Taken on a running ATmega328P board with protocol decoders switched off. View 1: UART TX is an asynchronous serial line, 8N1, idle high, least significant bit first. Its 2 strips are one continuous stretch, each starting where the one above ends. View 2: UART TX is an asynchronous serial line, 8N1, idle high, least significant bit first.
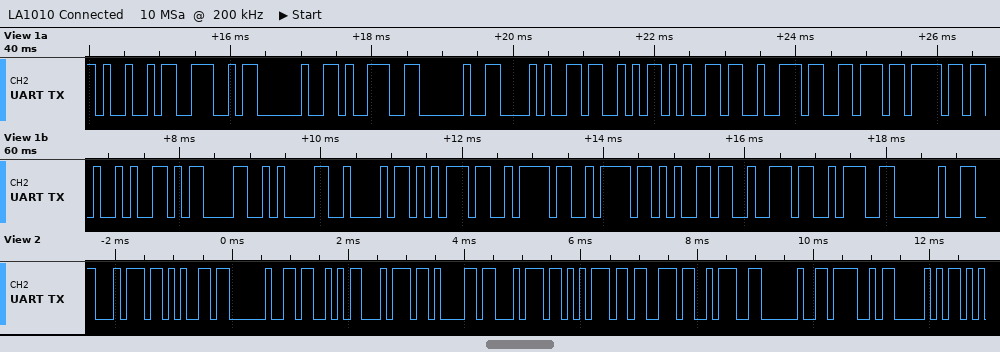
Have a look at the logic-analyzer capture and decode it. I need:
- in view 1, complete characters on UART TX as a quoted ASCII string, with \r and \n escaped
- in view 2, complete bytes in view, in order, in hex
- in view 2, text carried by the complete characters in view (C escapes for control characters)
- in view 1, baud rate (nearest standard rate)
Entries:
"IN 9 (Servo)\r\nBuzzer: "
74 65 20 53 74 61 74 75 73 3A 20 4F 50
"te Status: OP"
9600 baud
